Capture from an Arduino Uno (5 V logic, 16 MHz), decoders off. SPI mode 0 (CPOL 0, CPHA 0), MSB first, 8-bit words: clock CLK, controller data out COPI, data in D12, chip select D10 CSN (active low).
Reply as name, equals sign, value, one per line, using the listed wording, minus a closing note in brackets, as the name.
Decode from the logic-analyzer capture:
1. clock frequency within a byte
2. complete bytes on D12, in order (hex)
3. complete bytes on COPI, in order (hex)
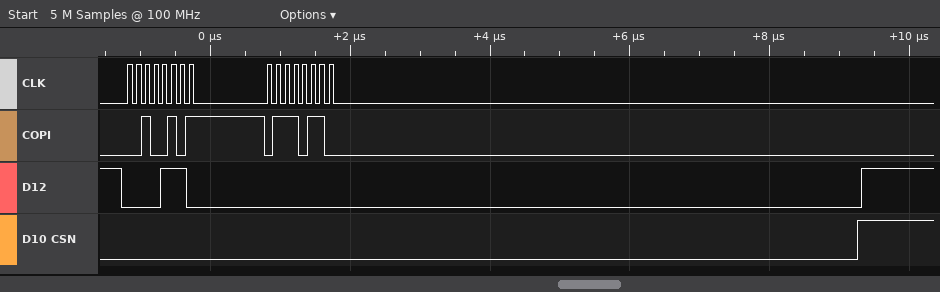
clock frequency within a byte = 8 MHz
complete bytes on D12, in order = 0E 00
complete bytes on COPI, in order = 25 76
